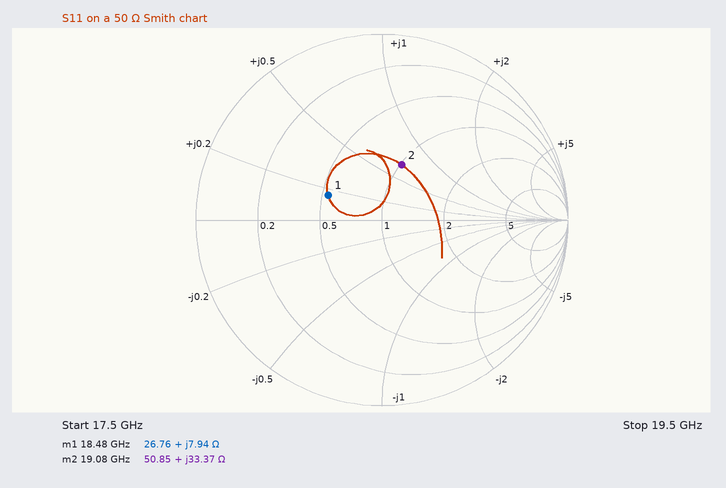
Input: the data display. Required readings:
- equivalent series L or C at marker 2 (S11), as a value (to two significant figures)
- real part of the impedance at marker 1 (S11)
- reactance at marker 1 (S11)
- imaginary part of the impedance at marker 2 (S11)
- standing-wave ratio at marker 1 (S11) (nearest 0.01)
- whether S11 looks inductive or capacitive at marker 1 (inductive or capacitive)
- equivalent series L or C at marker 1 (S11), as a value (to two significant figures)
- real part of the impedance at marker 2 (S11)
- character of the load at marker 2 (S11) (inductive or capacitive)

280 pH
26.76 Ω
+7.94 Ω
+33.37 Ω
1.93
inductive
68 pH
50.85 Ω
inductive
